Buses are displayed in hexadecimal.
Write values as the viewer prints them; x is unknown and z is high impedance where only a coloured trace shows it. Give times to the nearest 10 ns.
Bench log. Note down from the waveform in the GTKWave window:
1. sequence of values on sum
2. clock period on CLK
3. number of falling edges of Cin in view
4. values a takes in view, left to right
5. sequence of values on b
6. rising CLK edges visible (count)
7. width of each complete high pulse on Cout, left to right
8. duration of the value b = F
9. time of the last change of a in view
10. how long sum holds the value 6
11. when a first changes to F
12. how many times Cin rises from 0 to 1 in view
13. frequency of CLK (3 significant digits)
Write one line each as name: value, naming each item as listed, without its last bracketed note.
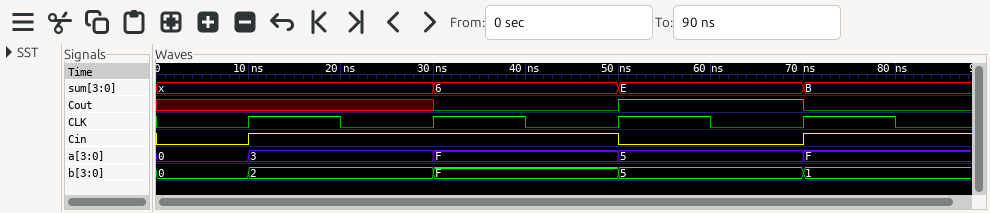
sequence of values on sum: x, 6, E, B
clock period on CLK: 20 ns
number of falling edges of Cin in view: 1
values a takes in view, left to right: 0, 3, F, 5, F
sequence of values on b: 0, 2, F, 5, 1
rising CLK edges visible: 4
width of each complete high pulse on Cout, left to right: 20 ns
duration of the value b = F: 20 ns
time of the last change of a in view: 70 ns
how long sum holds the value 6: 20 ns
when a first changes to F: 30 ns
how many times Cin rises from 0 to 1 in view: 2
frequency of CLK: 50.0 MHz
